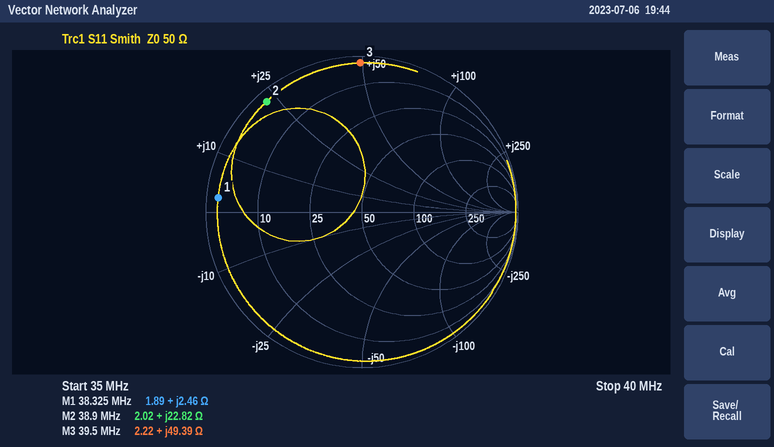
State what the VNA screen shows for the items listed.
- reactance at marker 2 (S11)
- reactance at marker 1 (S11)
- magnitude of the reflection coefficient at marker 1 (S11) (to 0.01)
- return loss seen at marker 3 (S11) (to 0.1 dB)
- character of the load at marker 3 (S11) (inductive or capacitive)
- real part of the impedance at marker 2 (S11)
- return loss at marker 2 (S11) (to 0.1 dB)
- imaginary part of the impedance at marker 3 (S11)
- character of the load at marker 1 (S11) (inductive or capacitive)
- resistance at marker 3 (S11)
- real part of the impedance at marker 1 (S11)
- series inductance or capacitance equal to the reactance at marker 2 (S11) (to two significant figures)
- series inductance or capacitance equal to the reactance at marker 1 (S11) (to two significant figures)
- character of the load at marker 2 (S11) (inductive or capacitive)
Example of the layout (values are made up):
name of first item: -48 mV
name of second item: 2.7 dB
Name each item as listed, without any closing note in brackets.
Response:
reactance at marker 2: +22.82 Ω
reactance at marker 1: +2.46 Ω
magnitude of the reflection coefficient at marker 1 (S11): 0.93
return loss seen at marker 3 (S11): 0.4 dB
character of the load at marker 3 (S11): inductive
real part of the impedance at marker 2: 2.02 Ω
return loss at marker 2 (S11): 0.6 dB
imaginary part of the impedance at marker 3: +49.39 Ω
character of the load at marker 1 (S11): inductive
resistance at marker 3: 2.22 Ω
real part of the impedance at marker 1: 1.89 Ω
series inductance or capacitance equal to the reactance at marker 2 (S11): 93 nH
series inductance or capacitance equal to the reactance at marker 1 (S11): 10 nH
character of the load at marker 2 (S11): inductive
